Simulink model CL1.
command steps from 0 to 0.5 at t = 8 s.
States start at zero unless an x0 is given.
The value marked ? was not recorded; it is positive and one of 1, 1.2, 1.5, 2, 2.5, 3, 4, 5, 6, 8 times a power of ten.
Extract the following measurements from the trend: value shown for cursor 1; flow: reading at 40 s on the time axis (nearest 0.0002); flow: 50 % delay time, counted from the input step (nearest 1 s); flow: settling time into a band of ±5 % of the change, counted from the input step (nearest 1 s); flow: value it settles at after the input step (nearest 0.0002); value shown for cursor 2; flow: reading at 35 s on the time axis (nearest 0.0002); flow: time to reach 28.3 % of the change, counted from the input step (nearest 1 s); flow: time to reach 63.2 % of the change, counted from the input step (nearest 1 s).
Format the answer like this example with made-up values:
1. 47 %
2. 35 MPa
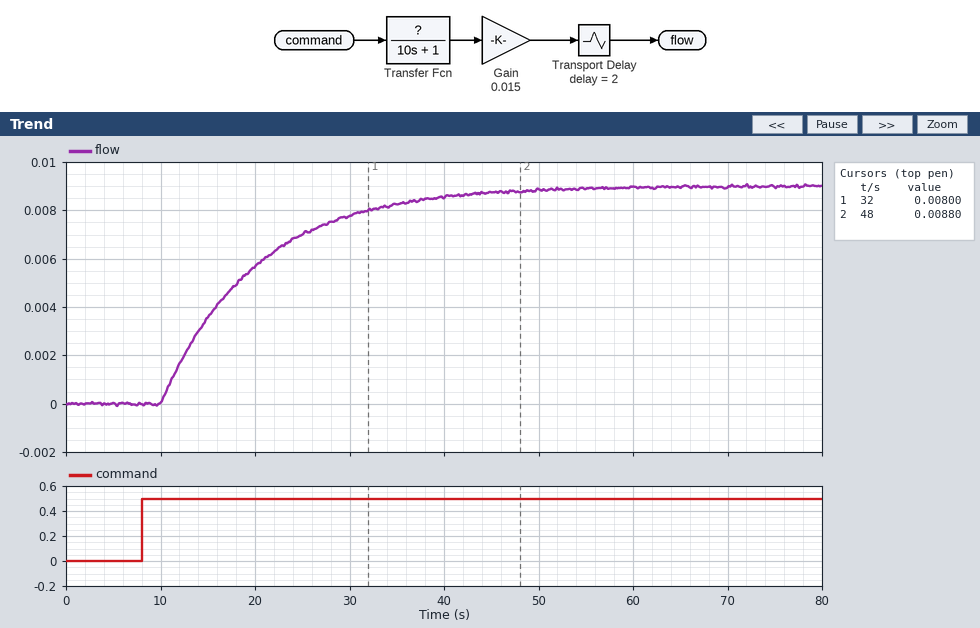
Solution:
1. 0.00800
2. 0.0086
3. 9 s
4. 32 s
5. 0.0090
6. 0.00880
7. 0.0082
8. 5 s
9. 12 s
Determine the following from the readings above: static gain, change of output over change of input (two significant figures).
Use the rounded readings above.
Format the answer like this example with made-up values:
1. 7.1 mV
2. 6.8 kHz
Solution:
1. 0.018
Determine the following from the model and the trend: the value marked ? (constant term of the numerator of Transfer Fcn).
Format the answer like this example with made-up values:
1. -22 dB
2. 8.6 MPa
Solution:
1. 1.2
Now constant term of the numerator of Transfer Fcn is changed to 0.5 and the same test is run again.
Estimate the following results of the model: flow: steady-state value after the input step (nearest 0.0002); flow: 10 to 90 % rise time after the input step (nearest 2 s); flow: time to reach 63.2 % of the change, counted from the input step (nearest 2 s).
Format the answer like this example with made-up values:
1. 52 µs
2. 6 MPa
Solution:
1. 0.0038
2. 22 s
3. 12 s
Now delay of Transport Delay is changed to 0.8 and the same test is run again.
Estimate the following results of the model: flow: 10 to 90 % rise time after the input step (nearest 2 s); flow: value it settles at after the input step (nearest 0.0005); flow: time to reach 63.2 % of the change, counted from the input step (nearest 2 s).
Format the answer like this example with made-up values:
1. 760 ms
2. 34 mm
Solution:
1. 22 s
2. 0.0090
3. 10 s
